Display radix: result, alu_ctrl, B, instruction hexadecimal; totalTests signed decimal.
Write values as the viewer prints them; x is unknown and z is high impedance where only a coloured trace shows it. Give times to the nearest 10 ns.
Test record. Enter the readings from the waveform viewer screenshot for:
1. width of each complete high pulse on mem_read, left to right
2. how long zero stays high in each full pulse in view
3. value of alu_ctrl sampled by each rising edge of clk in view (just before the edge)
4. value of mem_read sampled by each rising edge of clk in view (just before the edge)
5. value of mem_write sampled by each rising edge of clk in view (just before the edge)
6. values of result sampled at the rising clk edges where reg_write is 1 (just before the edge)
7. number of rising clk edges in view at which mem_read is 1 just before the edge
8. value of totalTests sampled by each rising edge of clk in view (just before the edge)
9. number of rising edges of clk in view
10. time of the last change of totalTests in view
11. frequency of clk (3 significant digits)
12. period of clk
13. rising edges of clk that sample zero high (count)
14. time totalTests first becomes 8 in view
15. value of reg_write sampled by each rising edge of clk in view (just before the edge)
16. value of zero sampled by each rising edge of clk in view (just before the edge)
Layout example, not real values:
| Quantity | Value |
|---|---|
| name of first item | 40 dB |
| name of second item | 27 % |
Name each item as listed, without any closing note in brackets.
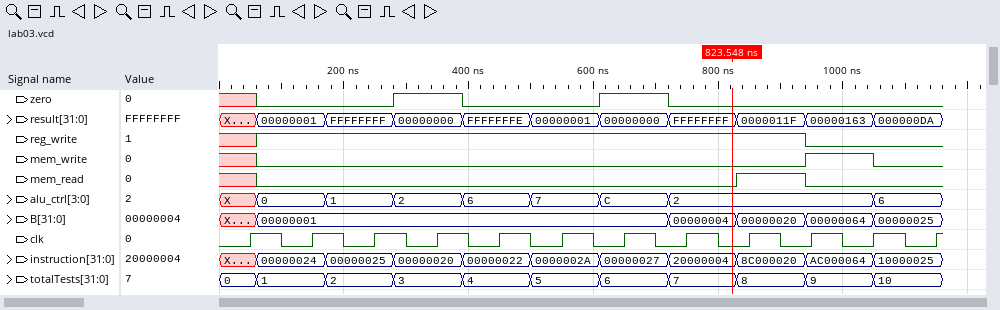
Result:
| Quantity | Value |
|---|---|
| width of each complete high pulse on mem_read, left to right | 110 ns |
| how long zero stays high in each full pulse in view | 110 ns, 110 ns |
| value of alu_ctrl sampled by each rising edge of clk in view | X, 0, 1, 2, 6, 7, C, 2, 2, 2, 2, 6 |
| value of mem_read sampled by each rising edge of clk in view | x 0 0 0 0 0 0 0 1 0 0 0 |
| value of mem_write sampled by each rising edge of clk in view | x 0 0 0 0 0 0 0 0 1 1 0 |
| values of result sampled at the rising clk edges where reg_write is 1 | 00000001, FFFFFFFF, 00000000, FFFFFFFE, 00000001, 00000000, FFFFFFFF, 0000011F |
| number of rising clk edges in view at which mem_read is 1 just before the edge | 1 |
| value of totalTests sampled by each rising edge of clk in view | 0, 1, 2, 3, 4, 5, 6, 7, 8, 9, 9, 10 |
| number of rising edges of clk in view | 12 |
| time of the last change of totalTests in view | 1050 ns |
| frequency of clk | 10.0 MHz |
| period of clk | 100 ns |
| rising edges of clk that sample zero high | 2 |
| time totalTests first becomes 8 in view | 830 ns |
| value of reg_write sampled by each rising edge of clk in view | x 1 1 1 1 1 1 1 1 0 0 0 |
| value of zero sampled by each rising edge of clk in view | x 0 0 1 0 0 1 0 0 0 0 0 |
